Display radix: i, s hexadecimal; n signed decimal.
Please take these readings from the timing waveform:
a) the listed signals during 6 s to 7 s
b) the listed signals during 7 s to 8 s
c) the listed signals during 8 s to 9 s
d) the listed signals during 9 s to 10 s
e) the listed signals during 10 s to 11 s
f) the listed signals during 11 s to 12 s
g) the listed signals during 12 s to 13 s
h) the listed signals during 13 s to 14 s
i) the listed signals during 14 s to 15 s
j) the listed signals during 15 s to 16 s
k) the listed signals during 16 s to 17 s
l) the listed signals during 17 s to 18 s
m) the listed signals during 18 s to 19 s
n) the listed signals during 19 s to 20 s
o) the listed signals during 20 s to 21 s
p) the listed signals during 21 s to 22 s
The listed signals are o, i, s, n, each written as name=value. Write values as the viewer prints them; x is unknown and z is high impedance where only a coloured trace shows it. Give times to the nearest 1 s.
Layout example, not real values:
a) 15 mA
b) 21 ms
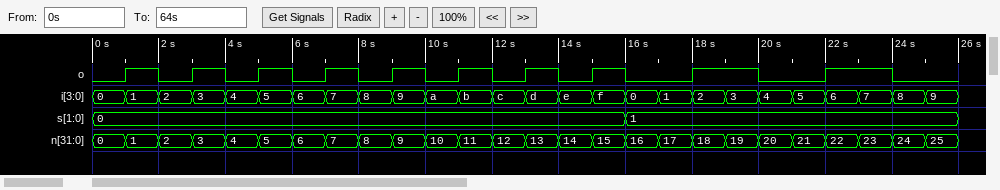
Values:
a) o=0, i=6, s=0, n=6
b) o=1, i=7, s=0, n=7
c) o=0, i=8, s=0, n=8
d) o=1, i=9, s=0, n=9
e) o=0, i=a, s=0, n=10
f) o=1, i=b, s=0, n=11
g) o=0, i=c, s=0, n=12
h) o=1, i=d, s=0, n=13
i) o=0, i=e, s=0, n=14
j) o=1, i=f, s=0, n=15
k) o=0, i=0, s=1, n=16
l) o=0, i=1, s=1, n=17
m) o=1, i=2, s=1, n=18
n) o=1, i=3, s=1, n=19
o) o=0, i=4, s=1, n=20
p) o=0, i=5, s=1, n=21
